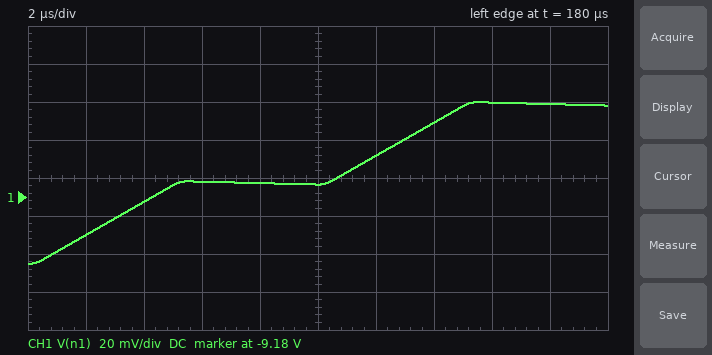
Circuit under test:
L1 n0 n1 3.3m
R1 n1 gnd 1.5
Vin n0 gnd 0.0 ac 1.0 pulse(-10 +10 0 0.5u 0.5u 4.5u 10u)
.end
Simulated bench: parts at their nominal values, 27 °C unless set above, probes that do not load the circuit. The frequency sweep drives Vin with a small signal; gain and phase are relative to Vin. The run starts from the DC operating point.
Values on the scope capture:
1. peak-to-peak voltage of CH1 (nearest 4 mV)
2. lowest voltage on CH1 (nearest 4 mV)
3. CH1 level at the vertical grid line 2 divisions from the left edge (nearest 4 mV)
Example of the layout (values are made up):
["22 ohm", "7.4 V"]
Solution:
["84 mV", "-9.216 V", "-9.184 V"]
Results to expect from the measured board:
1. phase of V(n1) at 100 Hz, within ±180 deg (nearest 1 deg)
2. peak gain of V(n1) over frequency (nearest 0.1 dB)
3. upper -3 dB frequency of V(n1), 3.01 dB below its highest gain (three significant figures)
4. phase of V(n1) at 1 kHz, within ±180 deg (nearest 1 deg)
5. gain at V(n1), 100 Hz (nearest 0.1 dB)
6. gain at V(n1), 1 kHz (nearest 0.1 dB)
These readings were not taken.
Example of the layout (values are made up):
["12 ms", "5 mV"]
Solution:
["-54 deg", "0 dB", "72.3 Hz", "-86 deg", "-4.6 dB", "-22.8 dB"]
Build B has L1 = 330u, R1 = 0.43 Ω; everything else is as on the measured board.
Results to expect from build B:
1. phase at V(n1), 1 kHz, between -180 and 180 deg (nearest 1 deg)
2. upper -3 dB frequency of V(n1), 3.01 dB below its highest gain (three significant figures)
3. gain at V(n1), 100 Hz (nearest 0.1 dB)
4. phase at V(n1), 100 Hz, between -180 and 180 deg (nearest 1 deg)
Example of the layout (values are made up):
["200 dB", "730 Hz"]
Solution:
["-78 deg", "207 Hz", "-0.9 dB", "-26 deg"]
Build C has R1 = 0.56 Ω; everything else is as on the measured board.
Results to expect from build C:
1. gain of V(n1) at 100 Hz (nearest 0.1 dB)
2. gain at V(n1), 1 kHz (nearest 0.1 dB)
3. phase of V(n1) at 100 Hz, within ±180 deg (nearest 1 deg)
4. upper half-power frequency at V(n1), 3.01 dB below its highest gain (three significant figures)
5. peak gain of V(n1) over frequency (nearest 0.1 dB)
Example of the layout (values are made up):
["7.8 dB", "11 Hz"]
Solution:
["-11.7 dB", "-31.4 dB", "-75 deg", "27.0 Hz", "0 dB"]
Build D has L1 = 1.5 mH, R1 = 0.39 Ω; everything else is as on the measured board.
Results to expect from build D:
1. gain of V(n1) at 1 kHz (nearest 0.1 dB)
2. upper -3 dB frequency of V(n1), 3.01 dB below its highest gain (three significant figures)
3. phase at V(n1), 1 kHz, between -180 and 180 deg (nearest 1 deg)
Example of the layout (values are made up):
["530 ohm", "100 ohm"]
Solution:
["-27.7 dB", "41.4 Hz", "-88 deg"]
